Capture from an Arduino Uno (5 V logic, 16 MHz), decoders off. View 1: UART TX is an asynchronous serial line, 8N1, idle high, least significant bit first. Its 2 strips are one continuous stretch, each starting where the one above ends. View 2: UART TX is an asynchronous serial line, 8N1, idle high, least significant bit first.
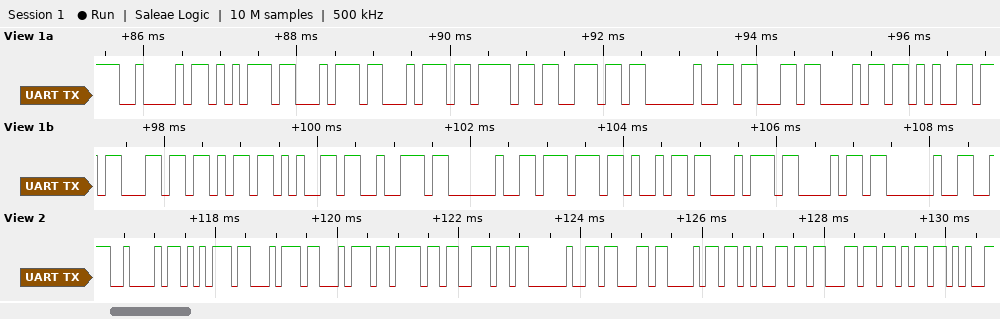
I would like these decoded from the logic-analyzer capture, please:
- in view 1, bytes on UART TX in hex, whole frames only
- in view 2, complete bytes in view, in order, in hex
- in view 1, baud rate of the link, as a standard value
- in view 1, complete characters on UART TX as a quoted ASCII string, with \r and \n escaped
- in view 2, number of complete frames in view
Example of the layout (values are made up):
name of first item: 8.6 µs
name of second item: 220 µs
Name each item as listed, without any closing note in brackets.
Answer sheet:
in view 1, bytes on UART TX in hex, whole frames only: 42 75 74 74 6F 6E 20 63 68 65 63 6B 65 72 20 77 69 74 68 20
in view 2, complete bytes in view, in order, in hex: 42 75 74 74 6F 6E 20 63 68 65 63 6B
in view 1, baud rate of the link, as a standard value: 9600 baud
in view 1, complete characters on UART TX as a quoted ASCII string, with \r and \n escaped: "Button checker with "
in view 2, number of complete frames in view: 12
